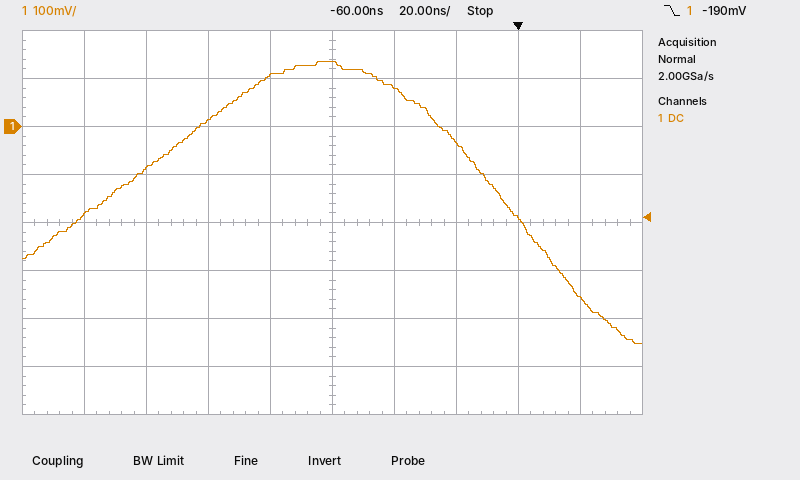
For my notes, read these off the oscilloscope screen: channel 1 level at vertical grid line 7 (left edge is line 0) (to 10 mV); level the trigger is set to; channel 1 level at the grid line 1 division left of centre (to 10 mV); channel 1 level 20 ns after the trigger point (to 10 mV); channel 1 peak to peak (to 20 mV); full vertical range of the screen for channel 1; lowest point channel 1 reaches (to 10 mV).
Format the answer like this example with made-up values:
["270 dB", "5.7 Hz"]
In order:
["-30 mV", "-190 mV", "110 mV", "-360 mV", "580 mV", "800 mV", "-450 mV"]
